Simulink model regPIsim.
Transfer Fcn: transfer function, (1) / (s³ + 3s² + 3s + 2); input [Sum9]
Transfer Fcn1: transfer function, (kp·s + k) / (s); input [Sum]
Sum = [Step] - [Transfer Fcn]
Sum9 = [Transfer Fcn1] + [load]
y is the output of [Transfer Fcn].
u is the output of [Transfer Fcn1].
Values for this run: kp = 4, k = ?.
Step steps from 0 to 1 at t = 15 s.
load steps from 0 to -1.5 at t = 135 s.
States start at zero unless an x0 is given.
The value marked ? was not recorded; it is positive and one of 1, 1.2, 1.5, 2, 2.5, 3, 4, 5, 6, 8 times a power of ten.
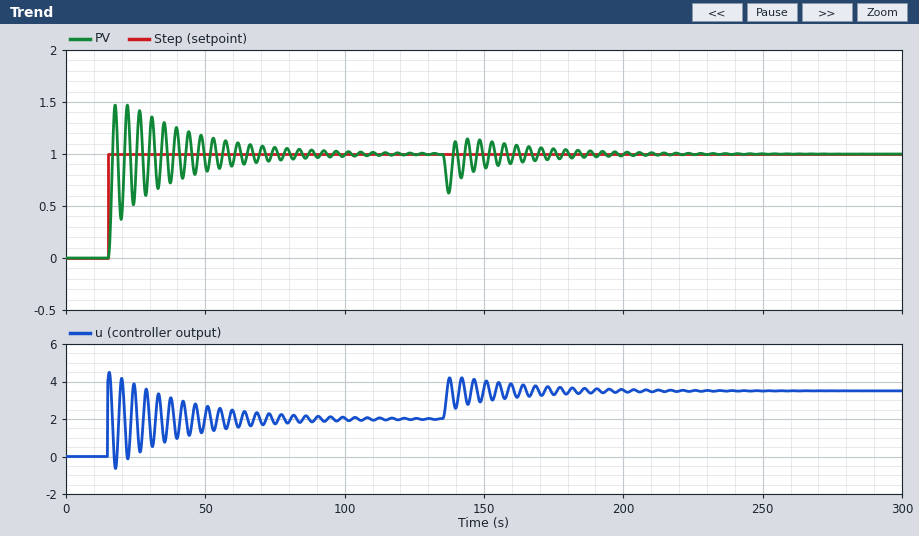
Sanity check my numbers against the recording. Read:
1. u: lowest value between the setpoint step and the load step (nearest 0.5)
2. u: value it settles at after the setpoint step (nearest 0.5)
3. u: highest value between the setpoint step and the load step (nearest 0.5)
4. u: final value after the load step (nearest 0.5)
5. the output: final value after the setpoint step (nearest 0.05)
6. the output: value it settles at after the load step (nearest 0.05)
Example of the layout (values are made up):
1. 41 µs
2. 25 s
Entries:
1. -0.5
2. 2.0
3. 4.5
4. 3.5
5. 1.00
6. 1.00
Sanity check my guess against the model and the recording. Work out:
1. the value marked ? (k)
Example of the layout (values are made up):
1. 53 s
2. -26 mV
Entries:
1. 1.5
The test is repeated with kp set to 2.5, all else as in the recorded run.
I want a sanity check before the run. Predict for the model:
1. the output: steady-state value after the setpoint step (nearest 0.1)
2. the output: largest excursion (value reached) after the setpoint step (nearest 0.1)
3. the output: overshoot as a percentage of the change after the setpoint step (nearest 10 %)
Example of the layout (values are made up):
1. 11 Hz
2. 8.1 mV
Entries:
1. 1.0
2. 1.4
3. 40 %
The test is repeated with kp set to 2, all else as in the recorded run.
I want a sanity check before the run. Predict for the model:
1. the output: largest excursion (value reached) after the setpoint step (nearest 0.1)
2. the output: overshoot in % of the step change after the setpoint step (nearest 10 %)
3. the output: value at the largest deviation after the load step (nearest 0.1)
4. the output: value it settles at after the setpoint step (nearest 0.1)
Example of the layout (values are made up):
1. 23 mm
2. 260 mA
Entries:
1. 1.4
2. 40 %
3. 0.5
4. 1.0
